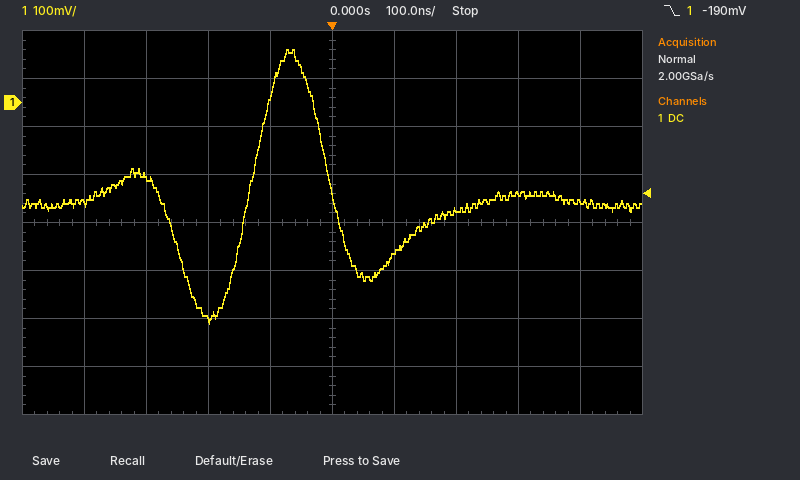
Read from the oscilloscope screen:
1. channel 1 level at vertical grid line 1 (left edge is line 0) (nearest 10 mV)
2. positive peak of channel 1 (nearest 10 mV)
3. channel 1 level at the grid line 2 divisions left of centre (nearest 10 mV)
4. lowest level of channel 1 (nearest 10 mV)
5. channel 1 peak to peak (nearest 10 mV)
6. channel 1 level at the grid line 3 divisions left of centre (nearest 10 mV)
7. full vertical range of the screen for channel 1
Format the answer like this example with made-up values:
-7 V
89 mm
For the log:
-210 mV
110 mV
-450 mV
-460 mV
570 mV
-150 mV
800 mV
